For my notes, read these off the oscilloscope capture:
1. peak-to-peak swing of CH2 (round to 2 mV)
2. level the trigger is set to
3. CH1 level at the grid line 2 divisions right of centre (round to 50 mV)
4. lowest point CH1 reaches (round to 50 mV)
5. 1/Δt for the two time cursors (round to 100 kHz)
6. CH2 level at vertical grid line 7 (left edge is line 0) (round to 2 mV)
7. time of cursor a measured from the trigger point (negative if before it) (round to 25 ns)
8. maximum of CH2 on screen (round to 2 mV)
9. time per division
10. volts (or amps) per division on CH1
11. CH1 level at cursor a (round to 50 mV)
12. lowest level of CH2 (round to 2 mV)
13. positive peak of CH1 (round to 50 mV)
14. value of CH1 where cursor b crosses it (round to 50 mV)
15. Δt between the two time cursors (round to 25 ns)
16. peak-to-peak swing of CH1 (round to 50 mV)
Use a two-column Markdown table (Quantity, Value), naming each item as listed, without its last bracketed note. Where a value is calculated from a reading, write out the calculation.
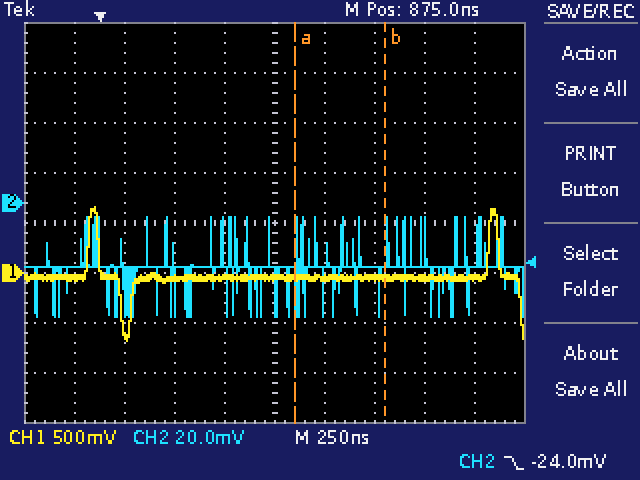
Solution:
| Quantity | Value |
|---|---|
| peak-to-peak swing of CH2 | -6 mV − (-46 mV) = 40 mV |
| level the trigger is set to | -24.0 mV |
| CH1 level at the grid line 2 divisions right of centre | -50 mV |
| lowest point CH1 reaches | -700 mV |
| 1/Δt for the two time cursors | 1 / 450 ns ≈ 2.2 MHz |
| CH2 level at vertical grid line 7 (left edge is line 0) | -26 mV |
| time of cursor a measured from the trigger point (negative if before it) | +975 ns |
| maximum of CH2 on screen | -6 mV |
| time per division | 250 ns |
| volts (or amps) per division on CH1 | 500 mV |
| CH1 level at cursor a | -50 mV |
| lowest level of CH2 | -46 mV |
| positive peak of CH1 | 650 mV |
| value of CH1 where cursor b crosses it | -50 mV |
| Δt between the two time cursors | 450 ns |
| peak-to-peak swing of CH1 | 650 mV − (-700 mV) = 1.35 V |
